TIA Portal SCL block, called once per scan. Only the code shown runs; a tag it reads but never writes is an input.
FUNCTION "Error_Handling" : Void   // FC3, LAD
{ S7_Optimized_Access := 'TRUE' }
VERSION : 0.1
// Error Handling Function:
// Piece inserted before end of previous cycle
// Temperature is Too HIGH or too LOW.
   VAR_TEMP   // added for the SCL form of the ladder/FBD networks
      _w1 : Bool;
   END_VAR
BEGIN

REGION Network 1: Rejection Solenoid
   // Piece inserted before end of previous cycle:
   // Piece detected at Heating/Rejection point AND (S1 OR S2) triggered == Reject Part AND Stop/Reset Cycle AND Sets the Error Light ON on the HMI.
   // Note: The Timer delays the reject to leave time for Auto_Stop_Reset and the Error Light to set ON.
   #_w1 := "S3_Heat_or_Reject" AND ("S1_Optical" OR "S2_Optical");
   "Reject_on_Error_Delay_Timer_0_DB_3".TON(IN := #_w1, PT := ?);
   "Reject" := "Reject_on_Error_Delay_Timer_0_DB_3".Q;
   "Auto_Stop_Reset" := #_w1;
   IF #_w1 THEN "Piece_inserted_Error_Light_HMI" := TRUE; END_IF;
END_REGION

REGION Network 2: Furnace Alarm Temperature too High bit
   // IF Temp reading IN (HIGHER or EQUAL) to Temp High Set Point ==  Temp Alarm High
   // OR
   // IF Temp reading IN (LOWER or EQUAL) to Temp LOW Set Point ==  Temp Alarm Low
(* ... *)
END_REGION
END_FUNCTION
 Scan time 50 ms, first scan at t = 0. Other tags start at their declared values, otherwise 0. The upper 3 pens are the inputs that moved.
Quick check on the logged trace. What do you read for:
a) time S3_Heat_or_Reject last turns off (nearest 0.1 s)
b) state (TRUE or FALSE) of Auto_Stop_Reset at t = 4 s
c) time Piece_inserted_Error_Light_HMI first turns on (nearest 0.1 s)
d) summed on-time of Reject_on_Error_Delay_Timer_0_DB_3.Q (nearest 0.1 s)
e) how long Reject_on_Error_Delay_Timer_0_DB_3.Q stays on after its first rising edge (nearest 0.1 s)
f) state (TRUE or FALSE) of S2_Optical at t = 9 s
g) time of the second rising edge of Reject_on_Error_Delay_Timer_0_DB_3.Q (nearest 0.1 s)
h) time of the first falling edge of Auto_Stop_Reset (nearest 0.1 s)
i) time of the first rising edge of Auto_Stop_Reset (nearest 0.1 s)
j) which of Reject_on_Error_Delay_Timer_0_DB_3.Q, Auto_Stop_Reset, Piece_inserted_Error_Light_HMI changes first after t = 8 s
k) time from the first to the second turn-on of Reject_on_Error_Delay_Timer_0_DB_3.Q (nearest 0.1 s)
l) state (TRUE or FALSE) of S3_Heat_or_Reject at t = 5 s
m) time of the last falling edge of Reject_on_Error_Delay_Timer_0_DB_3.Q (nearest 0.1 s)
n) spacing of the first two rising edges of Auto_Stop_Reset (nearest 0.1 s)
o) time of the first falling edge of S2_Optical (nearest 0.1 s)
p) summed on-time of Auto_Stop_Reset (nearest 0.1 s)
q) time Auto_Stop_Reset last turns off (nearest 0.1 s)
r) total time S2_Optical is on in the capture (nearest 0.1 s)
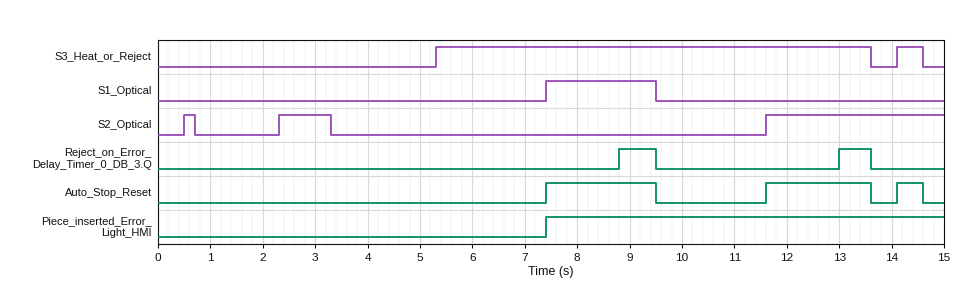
14.6 s
FALSE
7.4 s
1.3 s
0.7 s
FALSE
13.0 s
9.5 s
7.4 s
Reject_on_Error_Delay_Timer_0_DB_3.Q
4.2 s
FALSE
13.6 s
4.2 s
0.7 s
4.6 s
14.6 s
4.6 s
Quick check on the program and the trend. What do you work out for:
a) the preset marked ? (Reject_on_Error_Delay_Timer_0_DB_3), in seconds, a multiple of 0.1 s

1.4 s
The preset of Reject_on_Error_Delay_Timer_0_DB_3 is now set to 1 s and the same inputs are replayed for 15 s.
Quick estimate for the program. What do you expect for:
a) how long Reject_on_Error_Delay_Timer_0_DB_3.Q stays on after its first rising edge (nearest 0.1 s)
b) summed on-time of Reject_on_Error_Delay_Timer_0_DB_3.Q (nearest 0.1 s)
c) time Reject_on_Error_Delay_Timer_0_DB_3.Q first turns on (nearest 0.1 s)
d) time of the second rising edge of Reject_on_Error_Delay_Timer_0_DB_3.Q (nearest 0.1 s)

1.1 s
2.1 s
8.4 s
12.6 s
